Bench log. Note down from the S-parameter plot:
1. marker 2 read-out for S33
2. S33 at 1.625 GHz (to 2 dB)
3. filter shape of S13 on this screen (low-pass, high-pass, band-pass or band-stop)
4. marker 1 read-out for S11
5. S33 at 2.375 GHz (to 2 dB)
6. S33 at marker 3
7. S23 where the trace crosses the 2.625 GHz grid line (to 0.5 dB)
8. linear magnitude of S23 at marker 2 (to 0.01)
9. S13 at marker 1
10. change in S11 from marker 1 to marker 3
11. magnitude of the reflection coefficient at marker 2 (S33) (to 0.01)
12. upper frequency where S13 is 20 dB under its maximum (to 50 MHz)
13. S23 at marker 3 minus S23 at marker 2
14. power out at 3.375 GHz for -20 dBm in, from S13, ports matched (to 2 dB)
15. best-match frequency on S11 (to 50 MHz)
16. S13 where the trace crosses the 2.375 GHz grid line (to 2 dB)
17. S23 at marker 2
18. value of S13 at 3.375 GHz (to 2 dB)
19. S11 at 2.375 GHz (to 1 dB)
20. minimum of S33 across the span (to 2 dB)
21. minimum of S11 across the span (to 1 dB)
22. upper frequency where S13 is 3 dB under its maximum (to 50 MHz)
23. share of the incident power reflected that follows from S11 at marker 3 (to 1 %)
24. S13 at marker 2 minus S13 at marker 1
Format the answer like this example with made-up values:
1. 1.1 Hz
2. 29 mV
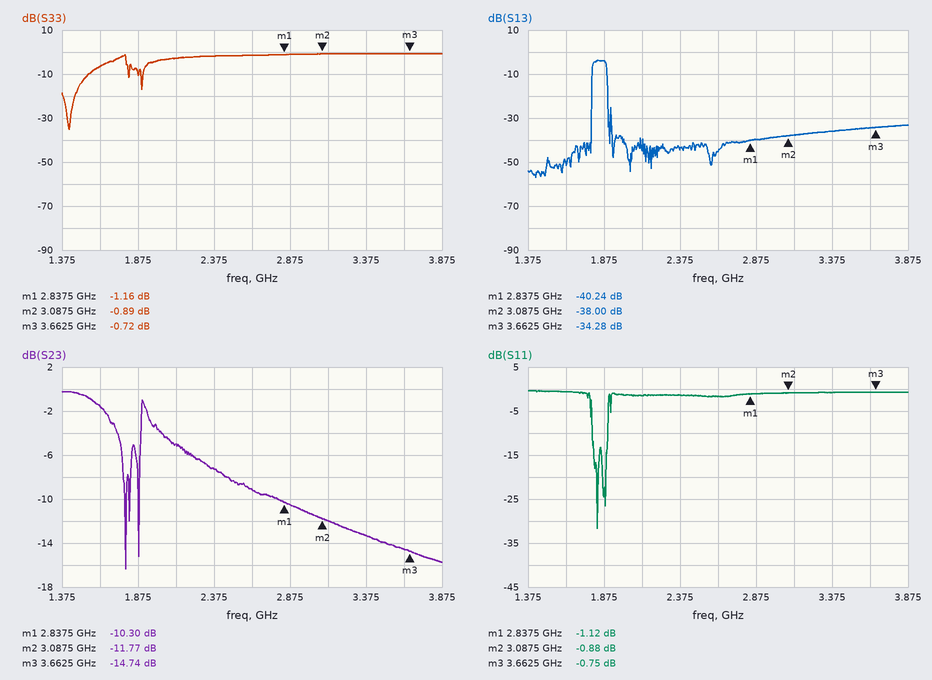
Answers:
1. -0.89 dB
2. -6 dB
3. band-pass
4. -1.12 dB
5. -2 dB
6. -0.72 dB
7. -9.0 dB
8. 0.26
9. -40.24 dB
10. 0.37 dB
11. 0.90
12. 1.90 GHz
13. -2.97 dB
14. -56 dBm
15. 1.85 GHz
16. -44 dB
17. -11.77 dB
18. -36 dB
19. -1 dB
20. -36 dB
21. -32 dB
22. 1.90 GHz
23. 84 %
24. 2.24 dB
